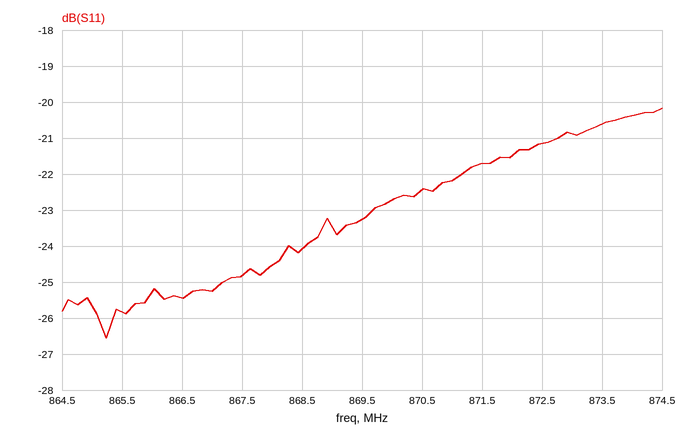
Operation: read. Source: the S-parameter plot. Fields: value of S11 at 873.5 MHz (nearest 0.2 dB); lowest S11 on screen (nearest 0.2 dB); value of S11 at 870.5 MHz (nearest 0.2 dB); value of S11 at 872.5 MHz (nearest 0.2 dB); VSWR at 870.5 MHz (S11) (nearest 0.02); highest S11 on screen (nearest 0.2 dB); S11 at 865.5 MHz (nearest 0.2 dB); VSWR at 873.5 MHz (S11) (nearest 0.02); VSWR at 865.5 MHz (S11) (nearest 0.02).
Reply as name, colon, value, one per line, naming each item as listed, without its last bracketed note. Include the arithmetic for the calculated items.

value of S11 at 873.5 MHz: -20.6 dB
lowest S11 on screen: -26.6 dB
value of S11 at 870.5 MHz: -22.4 dB
value of S11 at 872.5 MHz: -21.2 dB
VSWR at 870.5 MHz (S11): |Γ| = 10^(-22.4/20) = 0.0759; VSWR = (1 + 0.0759)/(1 − 0.0759) ≈ 1.16
highest S11 on screen: -20.2 dB
S11 at 865.5 MHz: -25.8 dB
VSWR at 873.5 MHz (S11): |Γ| = 10^(-20.6/20) = 0.0933; VSWR = (1 + 0.0933)/(1 − 0.0933) ≈ 1.21, so 1.20 to the nearest 0.02
VSWR at 865.5 MHz (S11): |Γ| = 10^(-25.8/20) = 0.0513; VSWR = (1 + 0.0513)/(1 − 0.0513) ≈ 1.11, so 1.10 to the nearest 0.02
